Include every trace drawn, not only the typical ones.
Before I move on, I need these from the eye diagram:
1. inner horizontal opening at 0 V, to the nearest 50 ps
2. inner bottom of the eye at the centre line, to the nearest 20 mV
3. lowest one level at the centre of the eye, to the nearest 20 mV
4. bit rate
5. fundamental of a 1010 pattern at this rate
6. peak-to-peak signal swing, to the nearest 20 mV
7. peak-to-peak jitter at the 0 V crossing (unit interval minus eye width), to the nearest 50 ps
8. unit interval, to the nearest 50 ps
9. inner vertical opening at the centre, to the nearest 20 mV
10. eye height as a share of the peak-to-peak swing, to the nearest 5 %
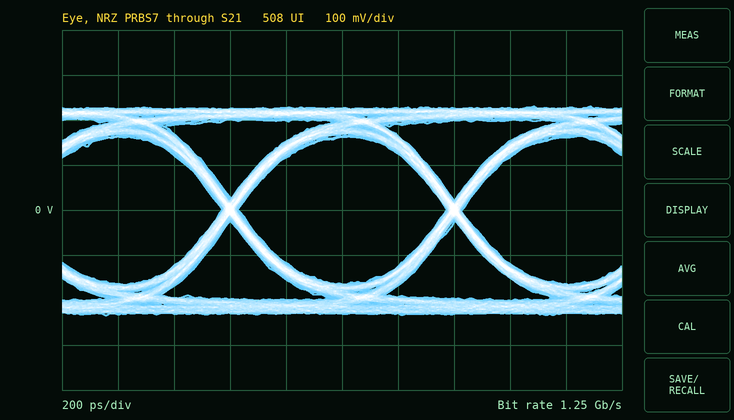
750 ps
-160 mV
160 mV
1.25 Gb/s
625 MHz
460 mV
50 ps
800 ps
320 mV
70 %
